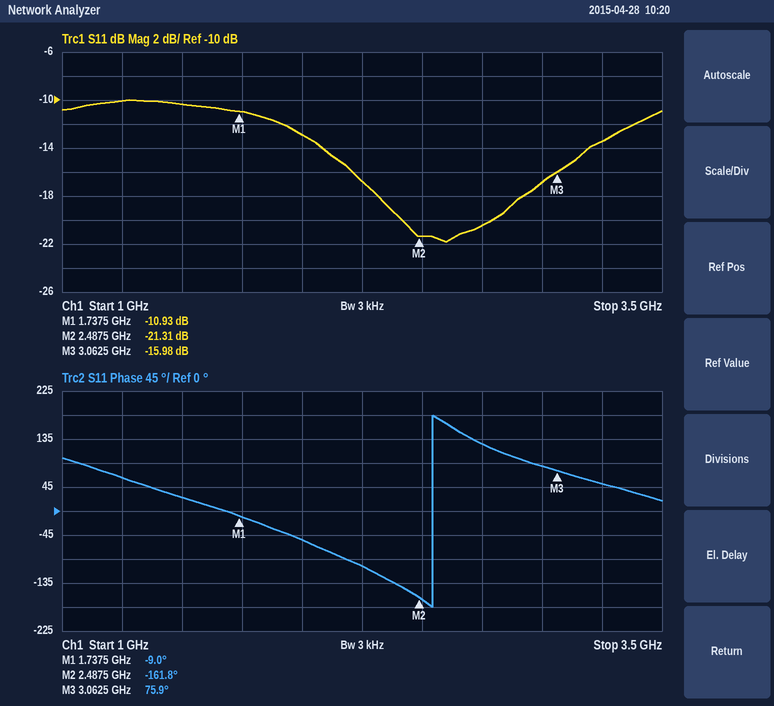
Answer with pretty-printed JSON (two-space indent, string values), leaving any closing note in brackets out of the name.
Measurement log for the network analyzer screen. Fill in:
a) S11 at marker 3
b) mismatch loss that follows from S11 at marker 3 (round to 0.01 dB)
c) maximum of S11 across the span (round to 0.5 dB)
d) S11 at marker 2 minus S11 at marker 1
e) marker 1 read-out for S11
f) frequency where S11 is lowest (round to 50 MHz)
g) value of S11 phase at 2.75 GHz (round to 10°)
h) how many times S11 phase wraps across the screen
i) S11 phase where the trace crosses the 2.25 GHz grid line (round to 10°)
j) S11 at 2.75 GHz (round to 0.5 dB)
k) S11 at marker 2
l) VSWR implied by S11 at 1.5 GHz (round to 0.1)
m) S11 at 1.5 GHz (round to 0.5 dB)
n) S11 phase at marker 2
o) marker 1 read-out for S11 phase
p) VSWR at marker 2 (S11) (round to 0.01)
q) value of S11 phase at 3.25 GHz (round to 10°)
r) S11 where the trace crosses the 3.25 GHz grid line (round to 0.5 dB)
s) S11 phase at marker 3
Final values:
{
  "S11 at marker 3": "-15.98 dB",
  "mismatch loss that follows from S11 at marker 3": "0.11 dB",
  "maximum of S11 across the span": "-10.0 dB",
  "S11 at marker 2 minus S11 at marker 1": "-10.38 dB",
  "marker 1 read-out for S11": "-10.93 dB",
  "frequency where S11 is lowest": "2.60 GHz",
  "value of S11 phase at 2.75 GHz": "130°",
  "how many times S11 phase wraps across the screen": "1",
  "S11 phase where the trace crosses the 2.25 GHz grid line": "-100°",
  "S11 at 2.75 GHz": "-20.5 dB",
  "S11 at marker 2": "-21.31 dB",
  "VSWR implied by S11 at 1.5 GHz": "1.9",
  "S11 at 1.5 GHz": "-10.5 dB",
  "S11 phase at marker 2": "-161.8°",
  "marker 1 read-out for S11 phase": "-9.0°",
  "VSWR at marker 2 (S11)": "1.19",
  "value of S11 phase at 3.25 GHz": "50°",
  "S11 where the trace crosses the 3.25 GHz grid line": "-13.5 dB",
  "S11 phase at marker 3": "75.9°"
}
